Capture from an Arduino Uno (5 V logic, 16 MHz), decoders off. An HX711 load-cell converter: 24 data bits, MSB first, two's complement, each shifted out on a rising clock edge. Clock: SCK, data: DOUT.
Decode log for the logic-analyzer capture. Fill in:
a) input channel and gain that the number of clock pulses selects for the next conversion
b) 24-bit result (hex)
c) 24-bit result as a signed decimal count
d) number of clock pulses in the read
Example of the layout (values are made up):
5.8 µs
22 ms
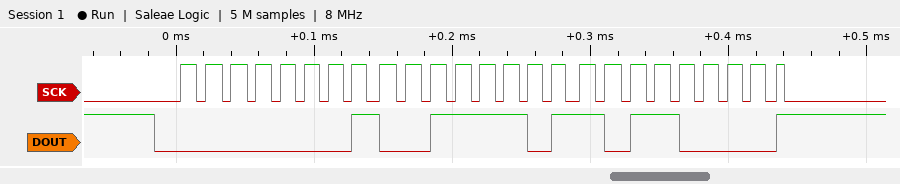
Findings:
channel A, gain 128
0x013DB0
81328
25
